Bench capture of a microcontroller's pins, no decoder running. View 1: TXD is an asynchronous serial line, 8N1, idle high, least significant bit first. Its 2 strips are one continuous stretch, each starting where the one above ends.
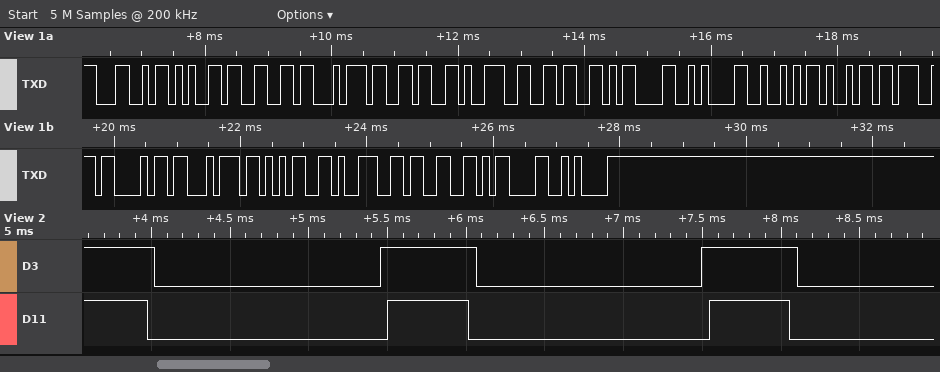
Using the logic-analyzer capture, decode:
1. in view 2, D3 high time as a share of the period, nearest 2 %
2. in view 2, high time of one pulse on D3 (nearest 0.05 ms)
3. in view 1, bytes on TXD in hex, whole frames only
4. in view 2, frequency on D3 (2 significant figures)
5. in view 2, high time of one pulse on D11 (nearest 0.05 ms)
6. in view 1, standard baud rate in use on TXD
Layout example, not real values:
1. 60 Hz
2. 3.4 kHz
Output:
1. 30 %
2. 0.60 ms
3. 4C 65 66 74 36 39 36 0D 0A 52 69 67 68 74 35 39 33 0D 0A
4. 490 Hz
5. 0.50 ms
6. 9600 baud
